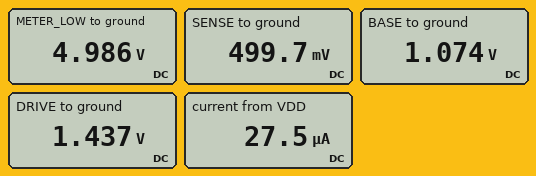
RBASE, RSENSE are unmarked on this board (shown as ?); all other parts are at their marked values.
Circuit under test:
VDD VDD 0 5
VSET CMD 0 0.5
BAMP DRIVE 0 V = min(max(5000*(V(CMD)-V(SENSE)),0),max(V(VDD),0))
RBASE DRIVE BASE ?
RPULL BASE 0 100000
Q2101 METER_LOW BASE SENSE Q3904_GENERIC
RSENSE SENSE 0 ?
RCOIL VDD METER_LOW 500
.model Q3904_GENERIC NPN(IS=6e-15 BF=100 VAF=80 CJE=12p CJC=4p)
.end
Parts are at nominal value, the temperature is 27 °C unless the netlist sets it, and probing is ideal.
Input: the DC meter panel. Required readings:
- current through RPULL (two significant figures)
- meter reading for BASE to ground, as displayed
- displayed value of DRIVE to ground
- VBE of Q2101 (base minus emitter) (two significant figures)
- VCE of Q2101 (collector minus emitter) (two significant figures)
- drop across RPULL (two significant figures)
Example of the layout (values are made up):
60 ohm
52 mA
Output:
11 µA
1.074 V
1.437 V
570 mV
4.5 V
1.1 V
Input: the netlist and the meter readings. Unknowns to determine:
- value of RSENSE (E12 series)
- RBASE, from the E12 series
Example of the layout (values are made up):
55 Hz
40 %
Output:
18 kΩ
33 kΩ
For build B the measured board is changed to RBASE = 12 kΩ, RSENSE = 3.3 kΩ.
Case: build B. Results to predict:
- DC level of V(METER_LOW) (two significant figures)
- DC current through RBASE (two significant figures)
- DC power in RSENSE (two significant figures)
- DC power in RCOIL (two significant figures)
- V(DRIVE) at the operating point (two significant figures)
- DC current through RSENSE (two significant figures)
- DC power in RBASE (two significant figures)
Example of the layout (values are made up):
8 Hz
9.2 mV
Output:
4.9 V
13 µA
76 µW
11 µW
1.3 V
150 µA
1.9 µW
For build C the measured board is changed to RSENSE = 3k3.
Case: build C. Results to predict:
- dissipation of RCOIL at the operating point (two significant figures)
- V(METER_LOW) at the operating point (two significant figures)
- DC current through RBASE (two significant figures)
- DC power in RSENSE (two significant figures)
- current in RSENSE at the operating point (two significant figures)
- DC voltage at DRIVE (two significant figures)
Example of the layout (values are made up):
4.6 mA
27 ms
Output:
11 µW
4.9 V
13 µA
76 µW
150 µA
1.5 V
